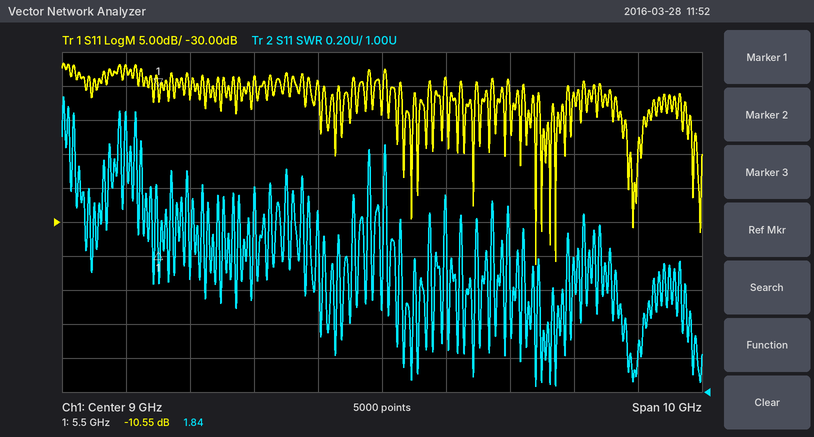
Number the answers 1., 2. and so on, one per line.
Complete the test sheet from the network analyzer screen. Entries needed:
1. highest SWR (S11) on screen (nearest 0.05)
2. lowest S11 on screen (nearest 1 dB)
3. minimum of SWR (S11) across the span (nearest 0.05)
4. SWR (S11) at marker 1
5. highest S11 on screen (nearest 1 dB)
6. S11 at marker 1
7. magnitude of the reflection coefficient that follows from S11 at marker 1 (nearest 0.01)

1. 2.75
2. -36 dB
3. 1.05
4. 1.84
5. -7 dB
6. -10.55 dB
7. 0.30
